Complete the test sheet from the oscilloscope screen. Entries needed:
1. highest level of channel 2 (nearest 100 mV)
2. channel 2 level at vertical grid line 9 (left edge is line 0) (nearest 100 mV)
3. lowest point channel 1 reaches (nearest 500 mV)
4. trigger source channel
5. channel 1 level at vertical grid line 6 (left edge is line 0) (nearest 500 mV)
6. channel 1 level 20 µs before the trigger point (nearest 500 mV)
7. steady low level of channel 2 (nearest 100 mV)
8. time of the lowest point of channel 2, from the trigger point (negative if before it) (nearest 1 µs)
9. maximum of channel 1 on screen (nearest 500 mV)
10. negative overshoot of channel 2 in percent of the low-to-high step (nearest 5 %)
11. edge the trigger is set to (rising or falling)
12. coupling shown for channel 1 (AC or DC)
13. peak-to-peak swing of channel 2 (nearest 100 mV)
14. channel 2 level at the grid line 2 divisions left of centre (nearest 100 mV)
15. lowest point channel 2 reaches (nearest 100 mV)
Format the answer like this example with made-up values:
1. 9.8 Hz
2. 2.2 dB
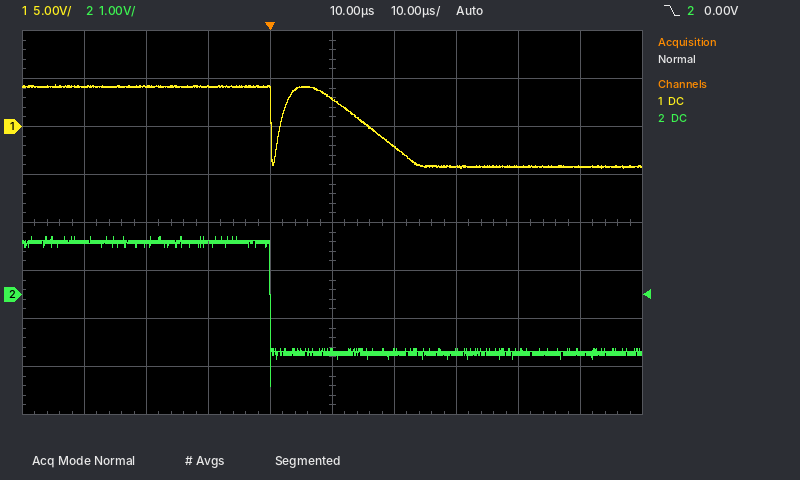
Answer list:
1. 1.2 V
2. -1.2 V
3. -4.5 V
4. channel 2
5. -2.0 V
6. 4.0 V
7. -1.2 V
8. 0 µs
9. 4.5 V
10. 30 %
11. falling
12. DC
13. 3.1 V
14. 1.1 V
15. -1.9 V
